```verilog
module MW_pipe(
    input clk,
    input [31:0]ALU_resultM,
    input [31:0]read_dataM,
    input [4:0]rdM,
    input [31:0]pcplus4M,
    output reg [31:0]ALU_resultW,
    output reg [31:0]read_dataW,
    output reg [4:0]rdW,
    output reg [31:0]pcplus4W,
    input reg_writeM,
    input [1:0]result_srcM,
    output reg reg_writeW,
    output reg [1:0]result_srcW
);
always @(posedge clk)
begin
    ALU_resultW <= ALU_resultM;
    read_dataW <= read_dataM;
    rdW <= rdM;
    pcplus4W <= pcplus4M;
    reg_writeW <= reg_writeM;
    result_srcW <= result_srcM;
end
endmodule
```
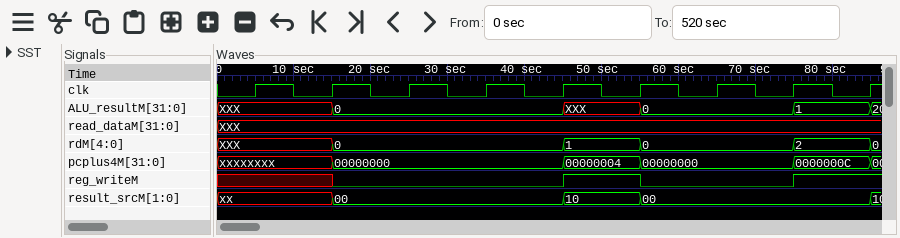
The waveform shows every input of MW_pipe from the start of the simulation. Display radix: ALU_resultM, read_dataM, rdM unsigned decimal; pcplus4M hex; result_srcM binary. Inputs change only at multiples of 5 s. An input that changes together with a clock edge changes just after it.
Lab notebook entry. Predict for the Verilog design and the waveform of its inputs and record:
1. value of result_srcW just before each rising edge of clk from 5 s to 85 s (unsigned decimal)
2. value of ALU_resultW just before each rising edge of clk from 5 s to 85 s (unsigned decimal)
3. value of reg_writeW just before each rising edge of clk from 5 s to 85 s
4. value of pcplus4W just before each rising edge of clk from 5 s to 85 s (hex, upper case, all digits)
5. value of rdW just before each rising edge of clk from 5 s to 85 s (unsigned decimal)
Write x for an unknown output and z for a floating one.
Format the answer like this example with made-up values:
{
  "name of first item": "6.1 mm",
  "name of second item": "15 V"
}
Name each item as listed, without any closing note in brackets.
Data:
{
  "value of result_srcW just before each rising edge of clk from 5 s to 85 s": "x, x, x, 0, 0, 0, 2, 0, 0",
  "value of ALU_resultW just before each rising edge of clk from 5 s to 85 s": "x, x, x, 0, 0, 0, x, 0, 0",
  "value of reg_writeW just before each rising edge of clk from 5 s to 85 s": "x x x 0 0 0 1 0 0",
  "value of pcplus4W just before each rising edge of clk from 5 s to 85 s": "x, x, x, 00000000, 00000000, 00000000, 00000004, 00000000, 00000000",
  "value of rdW just before each rising edge of clk from 5 s to 85 s": "x, x, x, 0, 0, 0, 1, 0, 0"
}
